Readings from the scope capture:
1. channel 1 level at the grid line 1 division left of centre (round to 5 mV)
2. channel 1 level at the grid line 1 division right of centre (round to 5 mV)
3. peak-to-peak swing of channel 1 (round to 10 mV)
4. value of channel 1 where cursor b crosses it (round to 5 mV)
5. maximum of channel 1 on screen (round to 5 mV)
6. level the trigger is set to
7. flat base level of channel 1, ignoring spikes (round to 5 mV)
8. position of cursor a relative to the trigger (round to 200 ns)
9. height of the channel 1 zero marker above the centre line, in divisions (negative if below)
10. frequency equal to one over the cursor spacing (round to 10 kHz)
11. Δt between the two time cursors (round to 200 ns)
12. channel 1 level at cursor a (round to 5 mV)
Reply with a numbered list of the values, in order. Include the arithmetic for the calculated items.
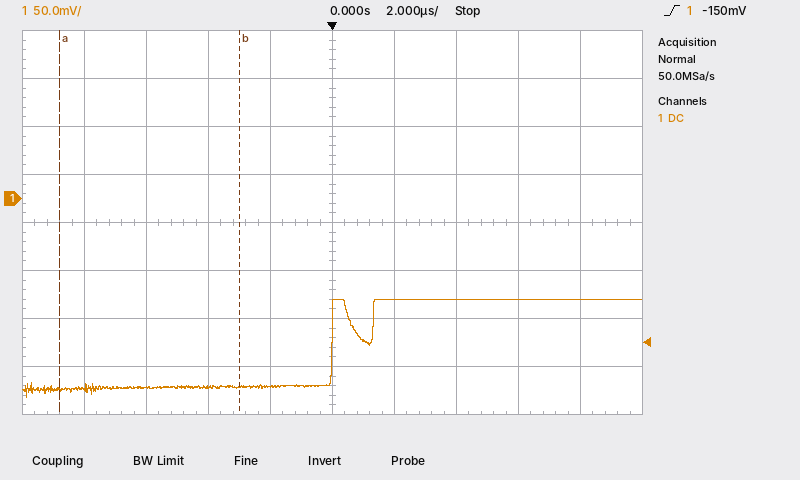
1. -195 mV
2. -105 mV
3. 100 mV
4. -195 mV
5. -105 mV
6. -150 mV
7. -195 mV
8. -8.8 µs
9. +0.5 div
10. 1 / 5.8 µs ≈ 170 kHz
11. 5.8 µs
12. -200 mV
